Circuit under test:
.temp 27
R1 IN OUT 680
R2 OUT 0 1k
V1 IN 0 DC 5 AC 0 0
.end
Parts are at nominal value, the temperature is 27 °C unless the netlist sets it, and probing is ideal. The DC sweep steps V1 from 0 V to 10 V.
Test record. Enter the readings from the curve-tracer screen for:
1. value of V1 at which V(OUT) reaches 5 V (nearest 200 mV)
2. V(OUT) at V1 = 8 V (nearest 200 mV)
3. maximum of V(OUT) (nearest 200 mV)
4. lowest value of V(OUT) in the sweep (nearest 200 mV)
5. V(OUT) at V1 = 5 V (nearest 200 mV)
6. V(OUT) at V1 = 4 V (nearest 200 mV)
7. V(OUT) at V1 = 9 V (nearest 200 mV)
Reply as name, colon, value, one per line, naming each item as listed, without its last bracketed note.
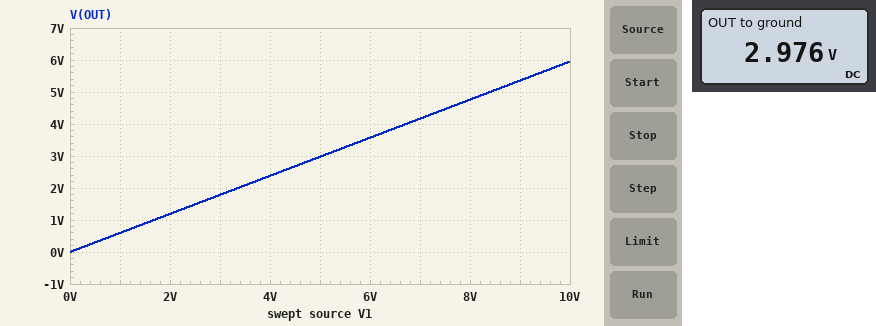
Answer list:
value of V1 at which V(OUT) reaches 5 V: 8.4 V
V(OUT) at V1 = 8 V: 4.8 V
maximum of V(OUT): 6.0 V
lowest value of V(OUT) in the sweep: 0 V
V(OUT) at V1 = 5 V: 3.0 V
V(OUT) at V1 = 4 V: 2.4 V
V(OUT) at V1 = 9 V: 5.4 V
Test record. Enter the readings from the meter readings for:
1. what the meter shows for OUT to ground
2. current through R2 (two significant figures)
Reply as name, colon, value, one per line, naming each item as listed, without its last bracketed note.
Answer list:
what the meter shows for OUT to ground: 2.976 V
current through R2: 3.0 mA
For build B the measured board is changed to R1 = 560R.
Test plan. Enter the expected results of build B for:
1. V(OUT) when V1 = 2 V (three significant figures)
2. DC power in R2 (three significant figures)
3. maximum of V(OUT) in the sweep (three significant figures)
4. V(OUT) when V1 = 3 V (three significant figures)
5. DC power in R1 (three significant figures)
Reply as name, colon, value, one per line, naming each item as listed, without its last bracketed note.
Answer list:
V(OUT) when V1 = 2 V: 1.28 V
DC power in R2: 10.3 mW
maximum of V(OUT) in the sweep: 6.41 V
V(OUT) when V1 = 3 V: 1.92 V
DC power in R1: 5.75 mW
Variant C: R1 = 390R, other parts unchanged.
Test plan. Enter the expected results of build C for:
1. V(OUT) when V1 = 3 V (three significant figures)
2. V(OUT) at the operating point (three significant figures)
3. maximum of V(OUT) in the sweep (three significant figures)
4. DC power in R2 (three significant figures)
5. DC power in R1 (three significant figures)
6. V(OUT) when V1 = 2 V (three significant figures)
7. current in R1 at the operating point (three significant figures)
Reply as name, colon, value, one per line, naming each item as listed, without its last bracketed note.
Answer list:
V(OUT) when V1 = 3 V: 2.16 V
V(OUT) at the operating point: 3.60 V
maximum of V(OUT) in the sweep: 7.19 V
DC power in R2: 12.9 mW
DC power in R1: 5.05 mW
V(OUT) when V1 = 2 V: 1.44 V
current in R1 at the operating point: 3.60 mA
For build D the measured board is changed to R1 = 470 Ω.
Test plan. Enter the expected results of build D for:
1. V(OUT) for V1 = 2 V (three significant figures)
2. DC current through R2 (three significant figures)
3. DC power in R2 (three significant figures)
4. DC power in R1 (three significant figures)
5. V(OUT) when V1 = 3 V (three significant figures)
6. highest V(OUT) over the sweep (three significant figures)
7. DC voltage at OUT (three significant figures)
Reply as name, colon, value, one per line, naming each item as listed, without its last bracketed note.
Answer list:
V(OUT) for V1 = 2 V: 1.36 V
DC current through R2: 3.40 mA
DC power in R2: 11.6 mW
DC power in R1: 5.44 mW
V(OUT) when V1 = 3 V: 2.04 V
highest V(OUT) over the sweep: 6.80 V
DC voltage at OUT: 3.40 V
